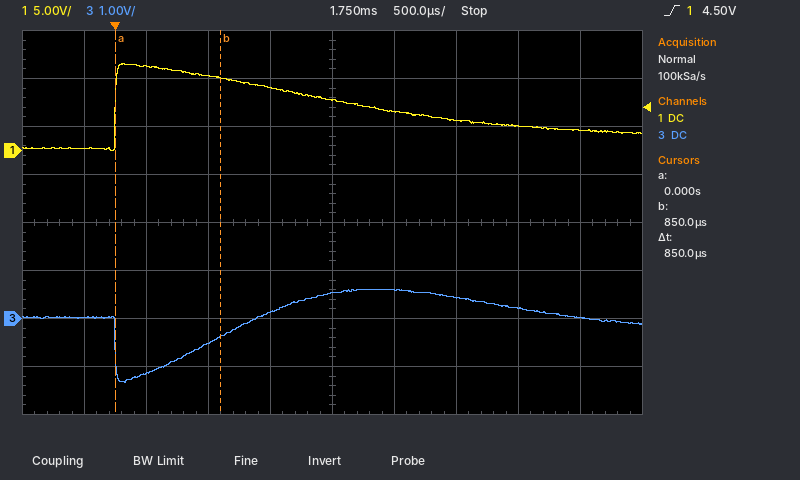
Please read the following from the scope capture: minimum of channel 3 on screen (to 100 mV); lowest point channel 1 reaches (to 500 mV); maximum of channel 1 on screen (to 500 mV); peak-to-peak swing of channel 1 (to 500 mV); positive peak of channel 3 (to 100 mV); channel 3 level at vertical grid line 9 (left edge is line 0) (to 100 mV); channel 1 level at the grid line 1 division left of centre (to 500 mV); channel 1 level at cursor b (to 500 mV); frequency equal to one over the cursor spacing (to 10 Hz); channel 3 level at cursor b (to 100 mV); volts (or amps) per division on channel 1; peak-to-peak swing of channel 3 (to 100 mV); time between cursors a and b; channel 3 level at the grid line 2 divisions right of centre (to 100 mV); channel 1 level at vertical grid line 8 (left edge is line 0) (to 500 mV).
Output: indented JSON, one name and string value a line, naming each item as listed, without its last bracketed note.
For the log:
{
  "minimum of channel 3 on screen": "-1.3 V",
  "lowest point channel 1 reaches": "0.0 V",
  "maximum of channel 1 on screen": "9.0 V",
  "peak-to-peak swing of channel 1": "9.0 V",
  "positive peak of channel 3": "600 mV",
  "channel 3 level at vertical grid line 9 (left edge is line 0)": "0.0 V",
  "channel 1 level at the grid line 1 division left of centre": "6.5 V",
  "channel 1 level at cursor b": "7.5 V",
  "frequency equal to one over the cursor spacing": "1.18 kHz",
  "channel 3 level at cursor b": "-400 mV",
  "volts (or amps) per division on channel 1": "5 V",
  "peak-to-peak swing of channel 3": "1.9 V",
  "time between cursors a and b": "850 µs",
  "channel 3 level at the grid line 2 divisions right of centre": "400 mV",
  "channel 1 level at vertical grid line 8 (left edge is line 0)": "2.5 V"
}
